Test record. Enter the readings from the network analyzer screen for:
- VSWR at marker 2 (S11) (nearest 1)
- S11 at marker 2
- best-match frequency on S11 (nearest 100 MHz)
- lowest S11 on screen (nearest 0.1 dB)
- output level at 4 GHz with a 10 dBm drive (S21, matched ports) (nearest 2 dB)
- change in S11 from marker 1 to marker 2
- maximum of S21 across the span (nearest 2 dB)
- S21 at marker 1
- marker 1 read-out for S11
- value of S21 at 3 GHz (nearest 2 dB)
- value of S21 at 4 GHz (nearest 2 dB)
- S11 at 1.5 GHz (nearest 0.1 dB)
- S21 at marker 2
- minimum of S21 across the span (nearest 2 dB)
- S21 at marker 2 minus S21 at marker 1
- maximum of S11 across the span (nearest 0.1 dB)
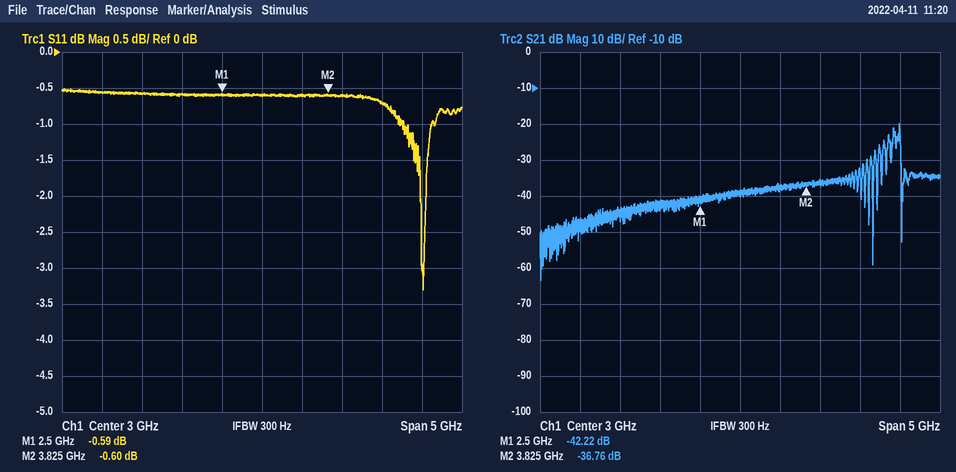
29
-0.60 dB
5.0 GHz
-3.3 dB
-26 dBm
-0.01 dB
-20 dB
-42.22 dB
-0.59 dB
-40 dB
-36 dB
-0.6 dB
-36.76 dB
-64 dB
5.46 dB
-0.5 dB
